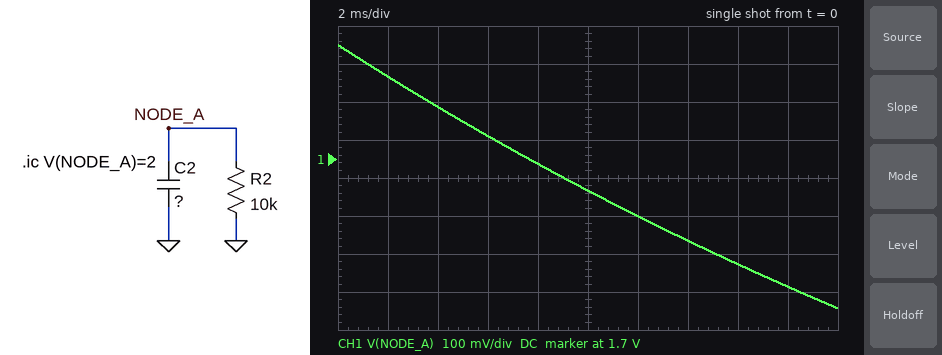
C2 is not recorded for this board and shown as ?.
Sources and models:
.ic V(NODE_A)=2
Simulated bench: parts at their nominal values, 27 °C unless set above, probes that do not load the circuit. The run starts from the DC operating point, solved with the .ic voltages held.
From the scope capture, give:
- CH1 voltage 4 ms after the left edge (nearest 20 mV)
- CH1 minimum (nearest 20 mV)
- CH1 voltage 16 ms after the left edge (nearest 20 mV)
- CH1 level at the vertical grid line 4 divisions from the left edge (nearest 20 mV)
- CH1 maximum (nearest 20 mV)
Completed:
1.84 V
1.30 V
1.42 V
1.68 V
2.00 V
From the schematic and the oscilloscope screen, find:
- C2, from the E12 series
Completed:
4.7 µF
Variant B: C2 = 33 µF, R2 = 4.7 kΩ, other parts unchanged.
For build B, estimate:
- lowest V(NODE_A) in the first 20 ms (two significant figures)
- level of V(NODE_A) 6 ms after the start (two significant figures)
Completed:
1.8 V
1.9 V
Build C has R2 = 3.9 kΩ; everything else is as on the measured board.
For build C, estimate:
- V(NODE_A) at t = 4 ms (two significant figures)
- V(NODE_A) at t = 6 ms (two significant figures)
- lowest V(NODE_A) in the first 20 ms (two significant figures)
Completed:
1.6 V
1.4 V
670 mV
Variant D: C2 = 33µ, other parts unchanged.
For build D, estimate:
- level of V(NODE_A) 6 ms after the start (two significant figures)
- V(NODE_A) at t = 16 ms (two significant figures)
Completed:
2.0 V
1.9 V
